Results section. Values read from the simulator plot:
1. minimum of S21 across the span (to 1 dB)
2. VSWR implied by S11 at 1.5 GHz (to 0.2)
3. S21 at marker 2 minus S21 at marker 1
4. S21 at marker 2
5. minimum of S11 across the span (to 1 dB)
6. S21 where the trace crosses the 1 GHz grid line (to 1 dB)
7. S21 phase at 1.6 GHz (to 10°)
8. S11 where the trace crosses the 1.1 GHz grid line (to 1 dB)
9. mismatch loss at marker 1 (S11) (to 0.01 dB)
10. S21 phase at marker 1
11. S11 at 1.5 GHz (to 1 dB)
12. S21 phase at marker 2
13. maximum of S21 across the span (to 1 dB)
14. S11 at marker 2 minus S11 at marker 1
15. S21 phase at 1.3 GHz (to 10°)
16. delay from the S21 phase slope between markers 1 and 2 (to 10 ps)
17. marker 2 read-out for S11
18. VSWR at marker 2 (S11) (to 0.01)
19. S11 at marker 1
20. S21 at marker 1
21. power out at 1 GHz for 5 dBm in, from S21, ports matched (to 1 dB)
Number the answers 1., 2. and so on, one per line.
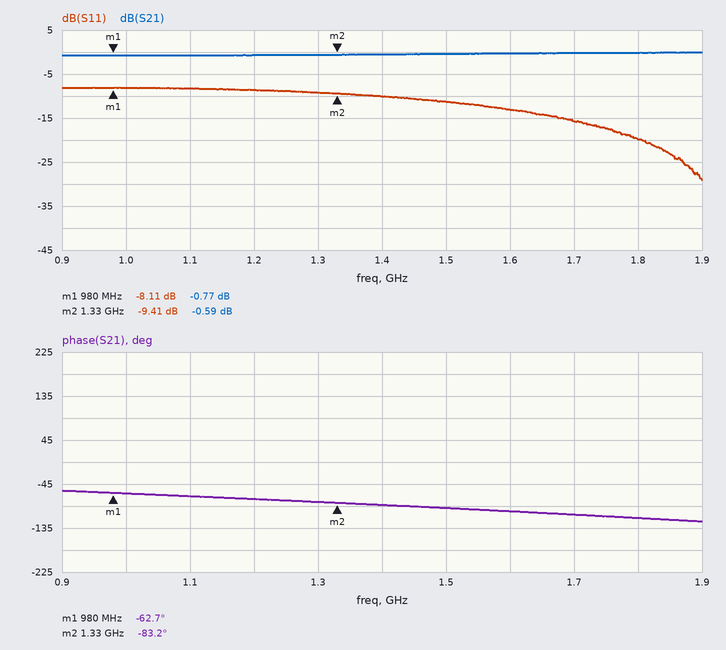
1. -1 dB
2. 1.8
3. 0.18 dB
4. -0.59 dB
5. -29 dB
6. -1 dB
7. -100°
8. -8 dB
9. 0.73 dB
10. -62.7°
11. -11 dB
12. -83.2°
13. 0 dB
14. -1.30 dB
15. -80°
16. 160 ps
17. -9.41 dB
18. 2.02
19. -8.11 dB
20. -0.77 dB
21. 4 dBm
